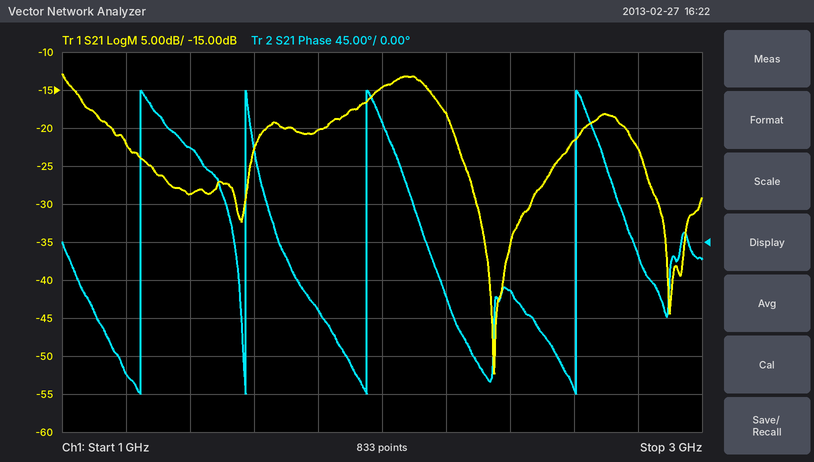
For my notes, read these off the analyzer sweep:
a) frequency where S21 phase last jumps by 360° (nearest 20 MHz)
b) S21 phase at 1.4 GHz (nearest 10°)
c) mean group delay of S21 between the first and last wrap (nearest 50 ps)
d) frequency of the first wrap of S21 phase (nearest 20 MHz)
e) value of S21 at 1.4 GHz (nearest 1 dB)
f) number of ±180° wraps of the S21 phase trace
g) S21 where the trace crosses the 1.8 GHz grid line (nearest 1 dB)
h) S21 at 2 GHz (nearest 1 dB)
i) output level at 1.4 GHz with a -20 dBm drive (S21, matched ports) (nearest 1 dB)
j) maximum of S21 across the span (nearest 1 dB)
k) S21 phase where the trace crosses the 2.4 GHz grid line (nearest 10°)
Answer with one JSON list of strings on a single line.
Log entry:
["2.60 GHz", "110°", "2.20 ns", "1.24 GHz", "-29 dB", "4", "-20 dB", "-15 dB", "-49 dBm", "-13 dB", "-60°"]
